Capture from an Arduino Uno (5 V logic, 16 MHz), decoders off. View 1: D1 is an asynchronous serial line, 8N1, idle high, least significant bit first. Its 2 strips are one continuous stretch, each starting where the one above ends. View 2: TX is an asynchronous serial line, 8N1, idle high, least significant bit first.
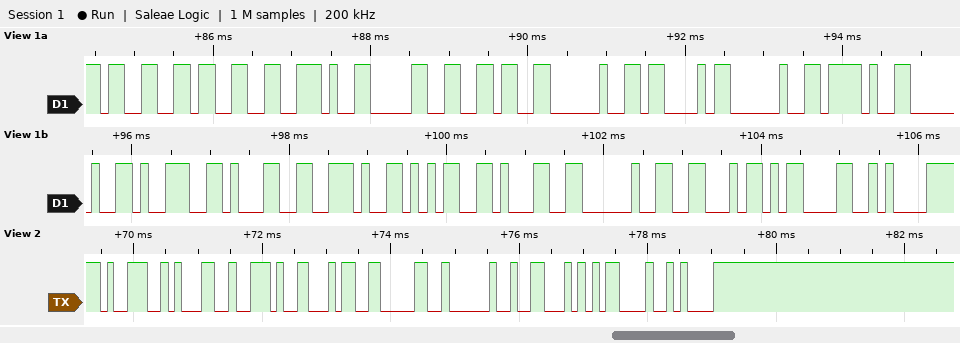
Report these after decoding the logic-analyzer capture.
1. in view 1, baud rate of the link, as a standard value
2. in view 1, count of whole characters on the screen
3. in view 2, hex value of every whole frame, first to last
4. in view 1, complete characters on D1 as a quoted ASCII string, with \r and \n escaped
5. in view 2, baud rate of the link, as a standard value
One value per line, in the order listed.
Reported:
9600 baud
19
0x39 0x31 0x2E 0x34 0x30 0x20 0x46 0x0D 0x0A
"33.06 C / 91.51 F\r\n"
9600 baud
